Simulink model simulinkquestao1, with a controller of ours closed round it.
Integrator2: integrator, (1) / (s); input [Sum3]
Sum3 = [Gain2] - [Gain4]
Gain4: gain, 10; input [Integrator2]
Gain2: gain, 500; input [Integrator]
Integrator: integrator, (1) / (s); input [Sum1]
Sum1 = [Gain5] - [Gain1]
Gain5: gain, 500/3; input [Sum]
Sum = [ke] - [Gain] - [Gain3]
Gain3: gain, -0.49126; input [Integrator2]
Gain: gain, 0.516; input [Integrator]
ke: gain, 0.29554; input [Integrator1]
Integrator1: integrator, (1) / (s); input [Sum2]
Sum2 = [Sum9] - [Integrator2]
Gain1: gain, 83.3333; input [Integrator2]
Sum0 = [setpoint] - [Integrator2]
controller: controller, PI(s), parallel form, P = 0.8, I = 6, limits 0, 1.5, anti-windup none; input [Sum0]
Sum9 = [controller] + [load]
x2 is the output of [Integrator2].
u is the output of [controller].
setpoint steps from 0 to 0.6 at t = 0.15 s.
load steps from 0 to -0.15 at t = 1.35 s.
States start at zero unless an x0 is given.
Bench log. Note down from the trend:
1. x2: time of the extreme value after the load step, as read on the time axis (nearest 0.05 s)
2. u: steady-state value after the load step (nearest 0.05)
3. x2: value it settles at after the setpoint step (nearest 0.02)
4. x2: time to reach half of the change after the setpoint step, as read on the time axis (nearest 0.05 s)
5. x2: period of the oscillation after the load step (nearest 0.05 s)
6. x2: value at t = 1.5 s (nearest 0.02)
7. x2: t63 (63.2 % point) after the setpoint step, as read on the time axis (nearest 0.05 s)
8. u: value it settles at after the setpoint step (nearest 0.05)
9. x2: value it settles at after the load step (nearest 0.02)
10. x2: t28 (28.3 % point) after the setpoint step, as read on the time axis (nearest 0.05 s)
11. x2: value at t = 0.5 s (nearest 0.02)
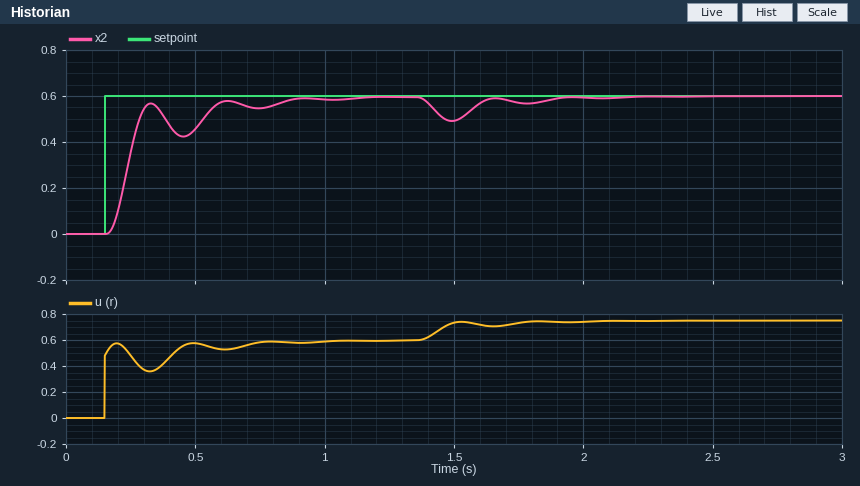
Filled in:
1.50 s
0.75
0.60
0.25 s
0.30 s
0.50
0.25 s
0.60
0.60
0.20 s
0.46
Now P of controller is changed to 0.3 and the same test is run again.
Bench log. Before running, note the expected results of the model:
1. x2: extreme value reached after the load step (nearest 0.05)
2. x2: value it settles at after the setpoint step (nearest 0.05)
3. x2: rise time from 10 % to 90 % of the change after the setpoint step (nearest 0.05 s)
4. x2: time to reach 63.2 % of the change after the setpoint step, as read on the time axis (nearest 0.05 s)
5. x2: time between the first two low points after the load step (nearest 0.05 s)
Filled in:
0.45
0.60
0.15 s
0.30 s
0.35 s
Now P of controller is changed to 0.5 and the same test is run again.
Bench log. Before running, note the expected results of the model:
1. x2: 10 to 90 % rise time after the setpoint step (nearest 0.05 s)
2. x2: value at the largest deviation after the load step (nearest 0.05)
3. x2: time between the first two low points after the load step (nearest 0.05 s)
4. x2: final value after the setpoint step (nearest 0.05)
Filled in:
0.15 s
0.50
0.35 s
0.60
